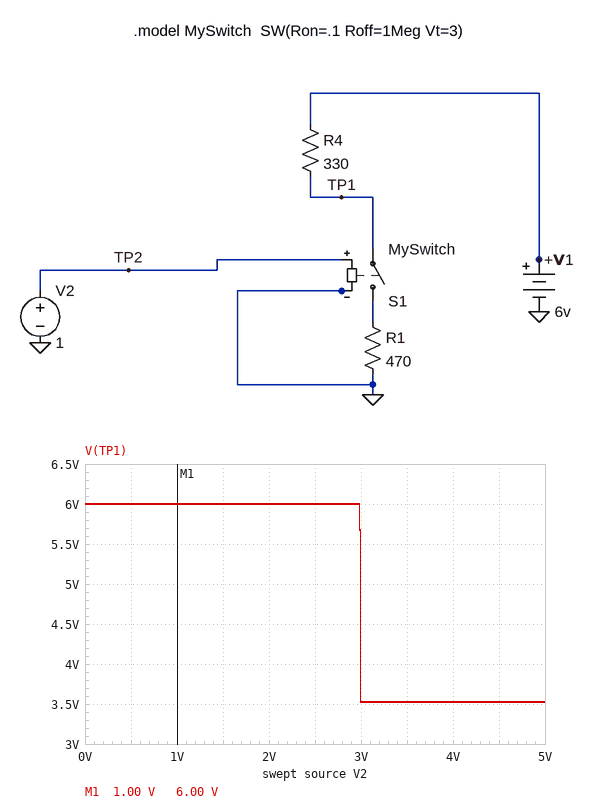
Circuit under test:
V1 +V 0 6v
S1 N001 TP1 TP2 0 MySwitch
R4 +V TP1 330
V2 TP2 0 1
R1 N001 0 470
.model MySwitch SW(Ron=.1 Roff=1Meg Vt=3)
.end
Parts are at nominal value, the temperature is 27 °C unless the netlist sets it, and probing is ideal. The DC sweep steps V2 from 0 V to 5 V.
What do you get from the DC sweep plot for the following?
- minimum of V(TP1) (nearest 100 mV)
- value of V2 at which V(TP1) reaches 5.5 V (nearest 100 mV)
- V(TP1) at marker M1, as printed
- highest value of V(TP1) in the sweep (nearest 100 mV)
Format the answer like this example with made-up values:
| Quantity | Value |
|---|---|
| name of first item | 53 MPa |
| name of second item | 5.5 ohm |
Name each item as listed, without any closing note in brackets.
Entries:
| Quantity | Value |
|---|---|
| minimum of V(TP1) | 3.5 V |
| value of V2 at which V(TP1) reaches 5.5 V | 3.0 V |
| V(TP1) at marker M1, as printed | 6.00 V |
| highest value of V(TP1) in the sweep | 6.0 V |
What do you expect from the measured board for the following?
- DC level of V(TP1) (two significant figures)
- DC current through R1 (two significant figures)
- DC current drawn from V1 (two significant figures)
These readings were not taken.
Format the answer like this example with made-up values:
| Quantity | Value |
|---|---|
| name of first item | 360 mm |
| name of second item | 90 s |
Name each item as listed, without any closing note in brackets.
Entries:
| Quantity | Value |
|---|---|
| DC level of V(TP1) | 6.0 V |
| DC current through R1 | 6.0 µA |
| DC current drawn from V1 | 6.0 µA |
